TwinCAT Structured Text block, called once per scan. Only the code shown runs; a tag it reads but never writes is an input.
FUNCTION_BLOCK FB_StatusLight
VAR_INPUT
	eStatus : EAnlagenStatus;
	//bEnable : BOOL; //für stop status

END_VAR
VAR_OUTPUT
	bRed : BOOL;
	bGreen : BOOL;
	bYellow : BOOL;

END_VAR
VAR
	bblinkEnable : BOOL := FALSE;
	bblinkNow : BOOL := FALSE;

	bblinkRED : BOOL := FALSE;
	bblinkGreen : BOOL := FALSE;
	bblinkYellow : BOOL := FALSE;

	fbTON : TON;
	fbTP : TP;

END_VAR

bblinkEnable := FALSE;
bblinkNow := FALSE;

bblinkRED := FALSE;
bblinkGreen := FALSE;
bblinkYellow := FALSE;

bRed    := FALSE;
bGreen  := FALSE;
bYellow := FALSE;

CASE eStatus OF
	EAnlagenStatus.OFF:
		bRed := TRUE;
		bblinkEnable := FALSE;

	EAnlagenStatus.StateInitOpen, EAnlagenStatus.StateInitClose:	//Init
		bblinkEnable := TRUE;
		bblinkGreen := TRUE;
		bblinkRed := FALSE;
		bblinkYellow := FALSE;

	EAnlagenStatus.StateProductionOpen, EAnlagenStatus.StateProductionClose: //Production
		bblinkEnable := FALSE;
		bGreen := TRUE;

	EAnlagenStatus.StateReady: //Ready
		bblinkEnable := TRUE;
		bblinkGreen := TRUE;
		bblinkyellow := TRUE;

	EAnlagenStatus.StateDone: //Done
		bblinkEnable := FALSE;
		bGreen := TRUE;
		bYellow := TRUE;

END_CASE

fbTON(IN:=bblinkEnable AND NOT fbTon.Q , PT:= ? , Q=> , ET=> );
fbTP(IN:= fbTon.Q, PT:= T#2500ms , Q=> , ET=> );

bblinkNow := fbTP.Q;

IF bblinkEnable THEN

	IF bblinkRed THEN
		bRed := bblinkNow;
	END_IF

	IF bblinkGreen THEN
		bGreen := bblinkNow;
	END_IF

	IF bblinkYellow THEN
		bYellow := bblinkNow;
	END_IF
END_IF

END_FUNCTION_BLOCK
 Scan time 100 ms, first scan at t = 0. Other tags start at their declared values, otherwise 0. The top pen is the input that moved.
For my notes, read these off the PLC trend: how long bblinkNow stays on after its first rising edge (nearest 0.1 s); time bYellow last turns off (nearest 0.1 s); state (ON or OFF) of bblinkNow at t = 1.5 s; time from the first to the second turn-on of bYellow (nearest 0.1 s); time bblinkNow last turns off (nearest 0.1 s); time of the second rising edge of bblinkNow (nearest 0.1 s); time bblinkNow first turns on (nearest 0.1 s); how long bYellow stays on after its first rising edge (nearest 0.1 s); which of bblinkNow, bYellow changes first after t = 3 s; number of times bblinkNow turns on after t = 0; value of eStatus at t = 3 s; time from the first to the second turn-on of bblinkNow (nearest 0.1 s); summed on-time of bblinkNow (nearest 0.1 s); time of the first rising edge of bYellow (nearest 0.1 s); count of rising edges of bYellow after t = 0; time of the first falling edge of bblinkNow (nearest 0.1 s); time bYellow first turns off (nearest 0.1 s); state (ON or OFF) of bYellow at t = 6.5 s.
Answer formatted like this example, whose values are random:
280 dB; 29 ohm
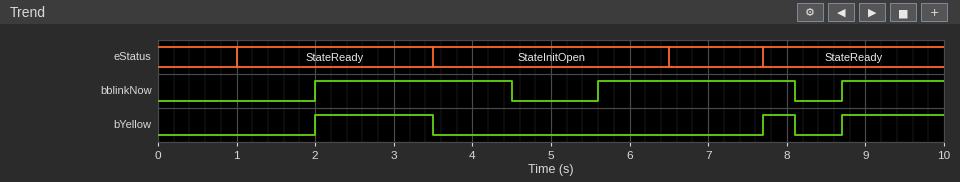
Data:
2.5 s; 8.1 s; OFF; 5.7 s; 8.1 s; 5.6 s; 2.0 s; 1.5 s; bYellow; 3; StateReady; 3.6 s; 6.3 s; 2.0 s; 3; 4.5 s; 3.5 s; OFF
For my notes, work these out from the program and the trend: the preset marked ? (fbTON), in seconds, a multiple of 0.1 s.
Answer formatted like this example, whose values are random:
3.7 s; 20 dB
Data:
1.0 s
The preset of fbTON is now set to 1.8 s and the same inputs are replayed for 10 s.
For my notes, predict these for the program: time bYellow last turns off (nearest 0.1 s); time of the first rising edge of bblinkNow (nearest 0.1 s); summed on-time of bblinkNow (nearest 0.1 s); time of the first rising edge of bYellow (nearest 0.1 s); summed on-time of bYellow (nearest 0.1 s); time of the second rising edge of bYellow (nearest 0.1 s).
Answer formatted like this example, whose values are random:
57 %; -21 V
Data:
3.5 s; 2.8 s; 3.0 s; 2.8 s; 1.2 s; 9.5 s
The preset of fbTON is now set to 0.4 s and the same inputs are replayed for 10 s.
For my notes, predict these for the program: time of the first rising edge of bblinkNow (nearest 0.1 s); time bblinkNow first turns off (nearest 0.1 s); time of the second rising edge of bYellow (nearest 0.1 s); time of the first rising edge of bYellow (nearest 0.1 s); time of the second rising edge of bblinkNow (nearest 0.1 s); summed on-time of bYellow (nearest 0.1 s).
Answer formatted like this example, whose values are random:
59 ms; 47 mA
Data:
1.4 s; 3.9 s; 8.1 s; 1.4 s; 4.4 s; 4.0 s
